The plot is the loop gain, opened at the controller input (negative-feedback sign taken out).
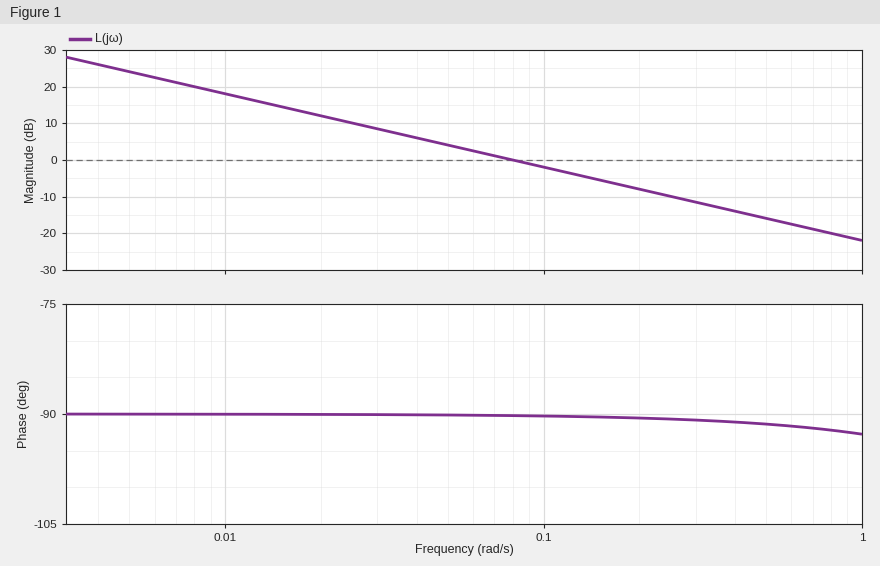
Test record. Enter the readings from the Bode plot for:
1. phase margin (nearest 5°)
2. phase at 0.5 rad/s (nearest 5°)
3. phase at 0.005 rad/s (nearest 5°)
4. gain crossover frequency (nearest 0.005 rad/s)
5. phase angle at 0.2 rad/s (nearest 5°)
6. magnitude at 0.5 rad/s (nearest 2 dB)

90°
-90°
-90°
0.080 rad/s
-90°
-16 dB
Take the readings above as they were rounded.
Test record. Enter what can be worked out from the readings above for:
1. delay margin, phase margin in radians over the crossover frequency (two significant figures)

20 s
